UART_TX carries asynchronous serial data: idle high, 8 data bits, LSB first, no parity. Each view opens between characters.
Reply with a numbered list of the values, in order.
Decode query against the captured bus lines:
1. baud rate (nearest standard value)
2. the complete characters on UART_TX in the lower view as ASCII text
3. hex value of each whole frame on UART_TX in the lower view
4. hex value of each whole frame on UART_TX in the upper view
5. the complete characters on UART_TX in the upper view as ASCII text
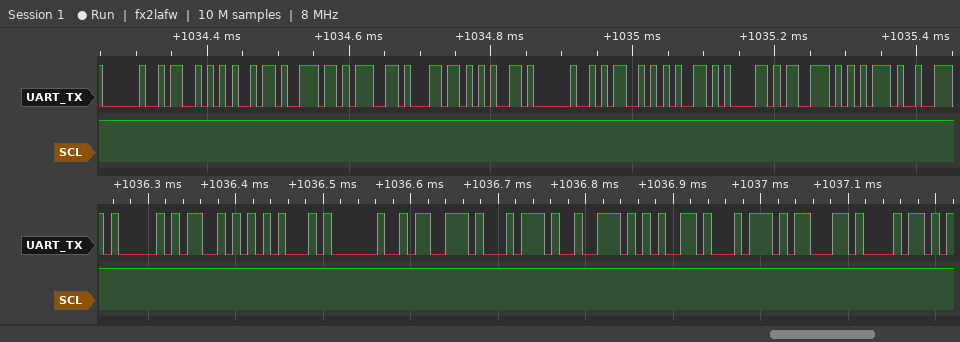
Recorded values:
1. 115200 baud
2. "ASE stretch"
3. 41, 53, 45, 20, 73, 74, 72, 65, 74, 63, 68
4. 20, 53, 69, 6E, 67, 6C, 65, 20, 4D, 65, 61, 73, 75
5. " Single Measu"
